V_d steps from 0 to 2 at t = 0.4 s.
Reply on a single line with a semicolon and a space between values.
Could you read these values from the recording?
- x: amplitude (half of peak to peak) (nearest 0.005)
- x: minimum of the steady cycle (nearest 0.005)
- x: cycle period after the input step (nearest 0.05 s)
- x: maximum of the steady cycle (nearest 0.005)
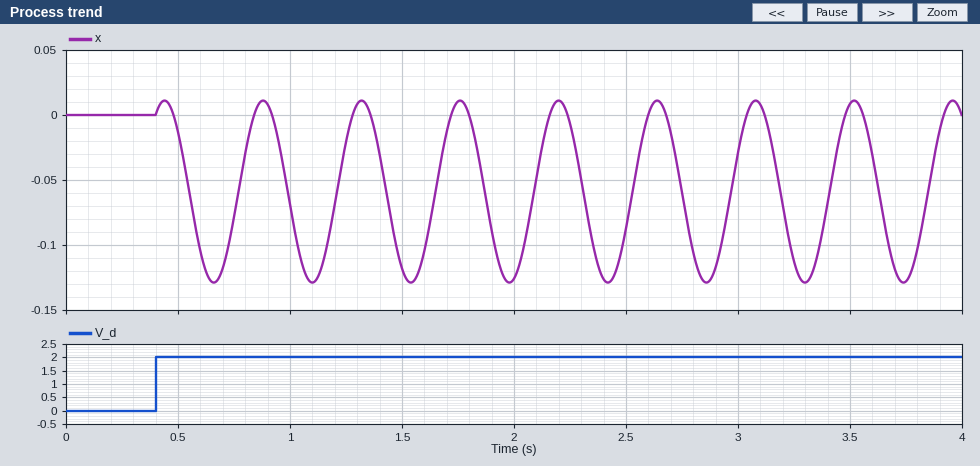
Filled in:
0.070; -0.130; 0.45 s; 0.010
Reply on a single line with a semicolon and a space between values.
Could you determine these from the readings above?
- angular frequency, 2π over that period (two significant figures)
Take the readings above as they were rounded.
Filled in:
14 rad/s
